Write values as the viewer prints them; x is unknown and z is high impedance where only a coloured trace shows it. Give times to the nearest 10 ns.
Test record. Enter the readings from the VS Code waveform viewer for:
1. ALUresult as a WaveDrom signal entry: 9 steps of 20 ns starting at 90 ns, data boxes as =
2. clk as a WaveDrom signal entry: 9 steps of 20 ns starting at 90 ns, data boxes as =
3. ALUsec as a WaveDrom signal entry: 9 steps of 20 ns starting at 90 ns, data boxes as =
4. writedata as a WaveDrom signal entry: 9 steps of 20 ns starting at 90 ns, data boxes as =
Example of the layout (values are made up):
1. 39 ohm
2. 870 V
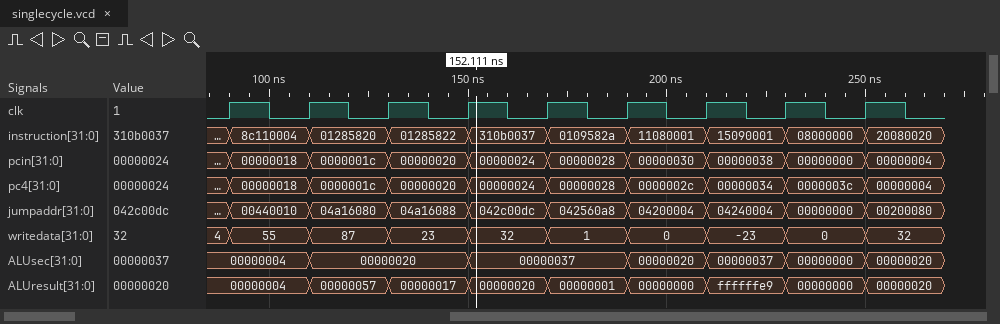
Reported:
1. {name: 'ALUresult', wave: '=========', data: '00000004 00000057 00000017 00000020 00000001 00000000 ffffffe9 00000000 00000020'}
2. {name: 'clk', wave: 'p........'}
3. {name: 'ALUsec', wave: '==.=.====', data: '00000004 00000020 00000037 00000020 00000037 00000000 00000020'}
4. {name: 'writedata', wave: '=========', data: '55 87 23 32 1 0 -23 0 32'}
